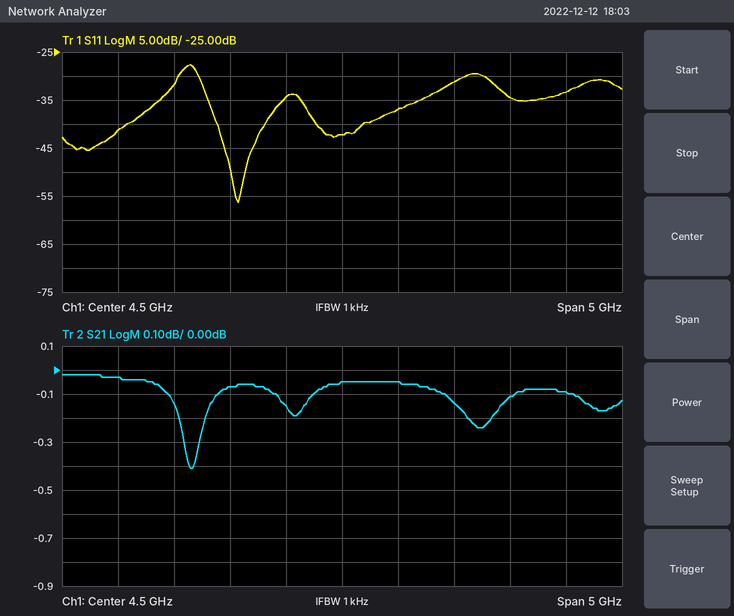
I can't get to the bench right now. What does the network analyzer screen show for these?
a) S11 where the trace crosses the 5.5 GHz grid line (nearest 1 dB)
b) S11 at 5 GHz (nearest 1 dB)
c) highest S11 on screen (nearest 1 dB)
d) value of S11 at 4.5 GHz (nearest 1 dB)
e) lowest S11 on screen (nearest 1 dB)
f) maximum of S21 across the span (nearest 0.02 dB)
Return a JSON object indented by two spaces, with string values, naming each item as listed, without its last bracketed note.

{
  "S11 where the trace crosses the 5.5 GHz grid line": "-31 dB",
  "S11 at 5 GHz": "-37 dB",
  "highest S11 on screen": "-28 dB",
  "value of S11 at 4.5 GHz": "-42 dB",
  "lowest S11 on screen": "-56 dB",
  "maximum of S21 across the span": "-0.02 dB"
}
